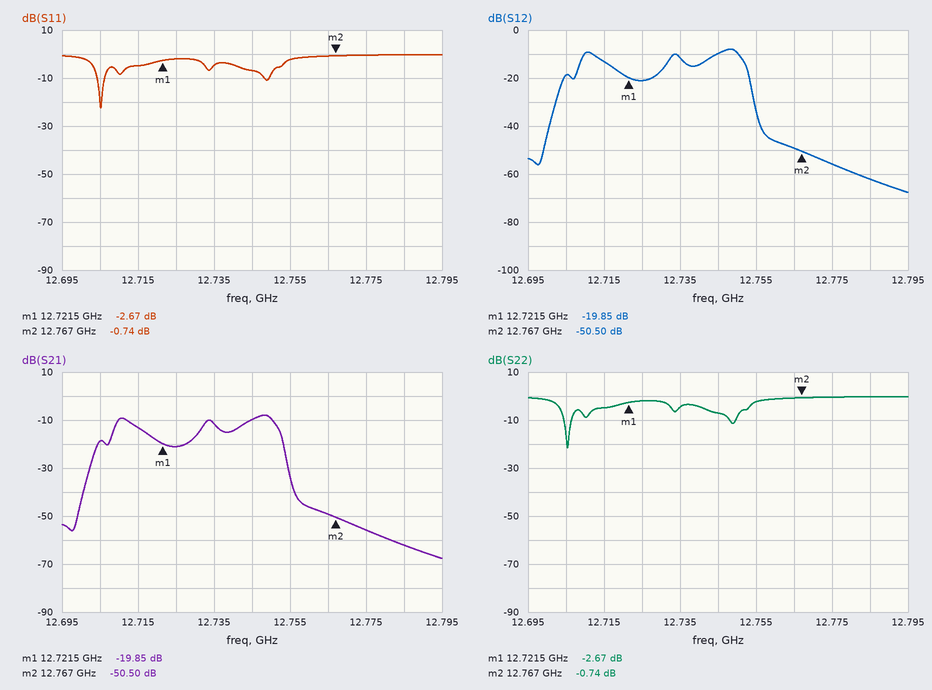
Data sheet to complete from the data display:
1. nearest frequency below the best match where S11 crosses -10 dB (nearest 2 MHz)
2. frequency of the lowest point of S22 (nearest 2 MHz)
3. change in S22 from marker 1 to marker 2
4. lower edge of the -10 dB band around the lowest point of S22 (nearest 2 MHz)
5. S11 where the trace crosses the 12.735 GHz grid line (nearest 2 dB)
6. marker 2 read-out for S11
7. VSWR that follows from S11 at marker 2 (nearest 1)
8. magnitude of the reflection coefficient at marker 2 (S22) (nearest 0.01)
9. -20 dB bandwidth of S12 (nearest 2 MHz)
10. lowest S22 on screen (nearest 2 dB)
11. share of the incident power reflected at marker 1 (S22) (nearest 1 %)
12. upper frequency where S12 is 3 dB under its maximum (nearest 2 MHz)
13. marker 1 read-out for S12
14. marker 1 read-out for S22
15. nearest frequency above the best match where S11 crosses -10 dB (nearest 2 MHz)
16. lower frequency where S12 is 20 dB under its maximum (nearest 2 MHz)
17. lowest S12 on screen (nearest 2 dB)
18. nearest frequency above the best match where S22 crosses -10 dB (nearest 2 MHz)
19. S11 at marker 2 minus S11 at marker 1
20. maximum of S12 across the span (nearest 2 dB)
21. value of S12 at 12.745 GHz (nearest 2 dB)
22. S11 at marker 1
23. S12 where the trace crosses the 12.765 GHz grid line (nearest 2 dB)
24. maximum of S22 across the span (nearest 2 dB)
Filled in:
12.704 GHz
12.706 GHz
1.93 dB
12.704 GHz
-4 dB
-0.74 dB
23
0.92
52 MHz
-22 dB
54 %
12.750 GHz
-19.85 dB
-2.67 dB
12.706 GHz
12.702 GHz
-68 dB
12.706 GHz
1.93 dB
-8 dB
-10 dB
-2.67 dB
-50 dB
0 dB
